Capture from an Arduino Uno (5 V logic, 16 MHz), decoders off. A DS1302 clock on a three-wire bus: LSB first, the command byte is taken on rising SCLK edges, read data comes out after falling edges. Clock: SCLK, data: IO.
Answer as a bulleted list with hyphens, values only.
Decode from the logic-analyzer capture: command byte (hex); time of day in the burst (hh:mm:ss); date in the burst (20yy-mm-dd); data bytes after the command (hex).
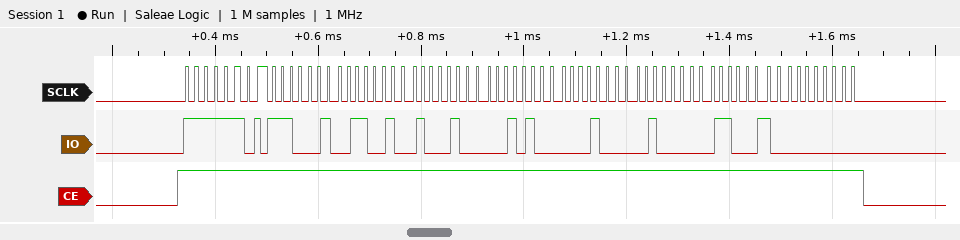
- 0xBF
- 11:26:47
- 2023-08-14
- 47 26 11 14 08 02 23 00
